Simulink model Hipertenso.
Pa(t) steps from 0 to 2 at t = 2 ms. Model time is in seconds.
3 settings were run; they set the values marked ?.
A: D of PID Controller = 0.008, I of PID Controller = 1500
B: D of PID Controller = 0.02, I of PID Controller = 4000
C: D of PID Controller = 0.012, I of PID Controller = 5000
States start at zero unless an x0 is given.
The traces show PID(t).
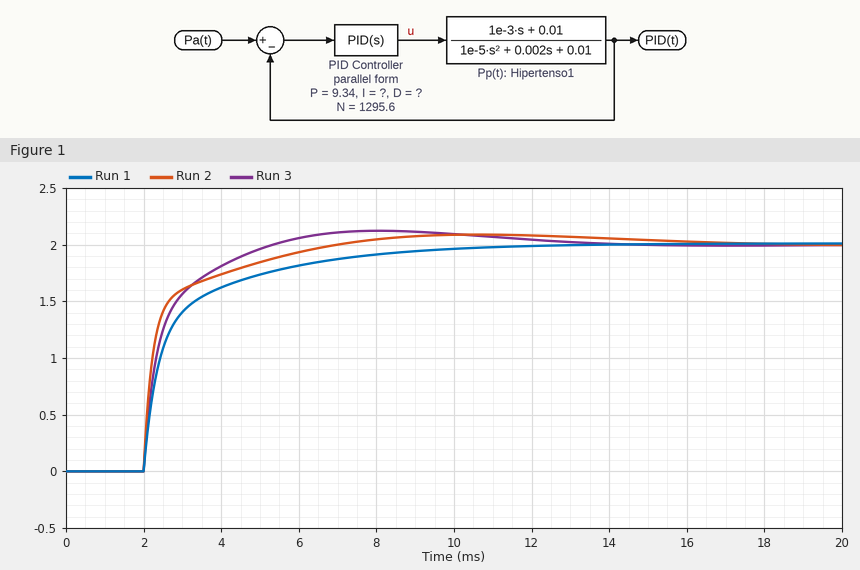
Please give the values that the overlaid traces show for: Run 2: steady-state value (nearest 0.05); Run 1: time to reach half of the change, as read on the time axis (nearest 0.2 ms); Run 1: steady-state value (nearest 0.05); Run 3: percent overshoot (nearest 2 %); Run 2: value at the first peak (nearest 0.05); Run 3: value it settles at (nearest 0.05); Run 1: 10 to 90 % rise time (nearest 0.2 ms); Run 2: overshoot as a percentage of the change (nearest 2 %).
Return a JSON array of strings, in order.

["2.00", "2.4 ms", "2.00", "6 %", "2.10", "2.00", "3.8 ms", "4 %"]
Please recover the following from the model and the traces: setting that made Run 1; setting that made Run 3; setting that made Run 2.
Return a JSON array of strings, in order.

["A", "C", "B"]
